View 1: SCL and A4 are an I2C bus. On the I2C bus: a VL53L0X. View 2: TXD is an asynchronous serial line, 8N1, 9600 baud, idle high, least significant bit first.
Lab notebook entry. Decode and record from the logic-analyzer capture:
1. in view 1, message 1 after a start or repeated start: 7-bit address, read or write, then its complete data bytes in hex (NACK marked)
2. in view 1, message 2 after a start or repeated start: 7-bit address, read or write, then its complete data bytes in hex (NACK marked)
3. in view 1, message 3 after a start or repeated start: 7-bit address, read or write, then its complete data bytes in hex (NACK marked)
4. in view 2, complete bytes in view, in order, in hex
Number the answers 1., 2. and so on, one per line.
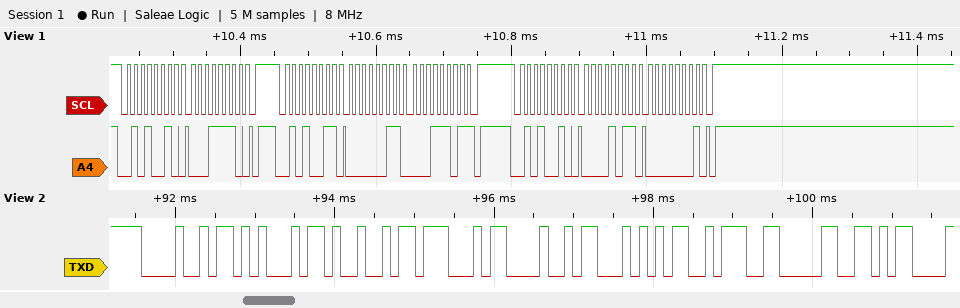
1. 0x29 write: 1E
2. 0x29 read: 03 1D NACK
3. 0x29 write: 0B 01
4. 48 45 49 47 48 54 3A 30 0D
